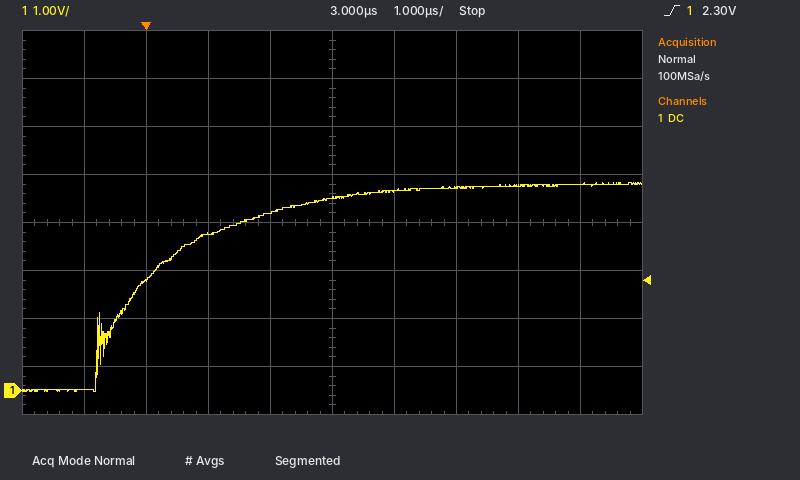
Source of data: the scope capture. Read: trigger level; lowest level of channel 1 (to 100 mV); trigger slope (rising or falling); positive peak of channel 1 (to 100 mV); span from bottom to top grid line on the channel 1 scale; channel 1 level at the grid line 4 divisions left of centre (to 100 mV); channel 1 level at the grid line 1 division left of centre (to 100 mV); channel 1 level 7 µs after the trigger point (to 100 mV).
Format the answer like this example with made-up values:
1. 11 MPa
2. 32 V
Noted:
1. 2.30 V
2. 0.0 V
3. rising
4. 4.3 V
5. 8 V
6. 0.0 V
7. 3.7 V
8. 4.3 V
